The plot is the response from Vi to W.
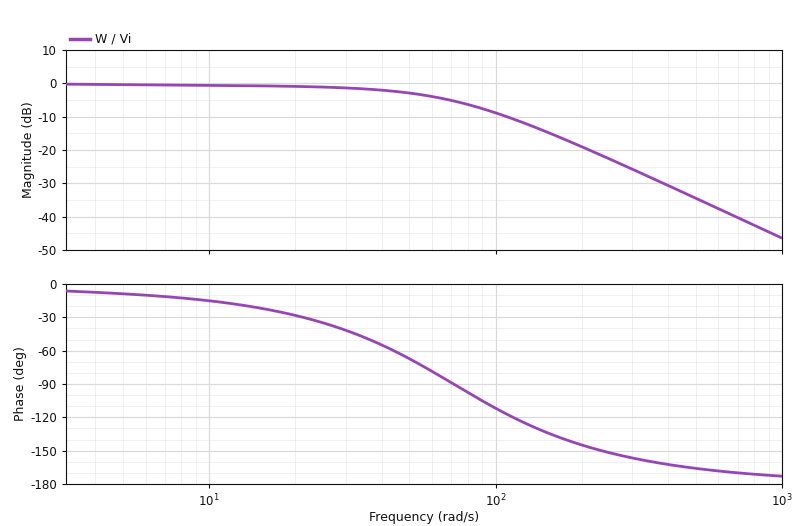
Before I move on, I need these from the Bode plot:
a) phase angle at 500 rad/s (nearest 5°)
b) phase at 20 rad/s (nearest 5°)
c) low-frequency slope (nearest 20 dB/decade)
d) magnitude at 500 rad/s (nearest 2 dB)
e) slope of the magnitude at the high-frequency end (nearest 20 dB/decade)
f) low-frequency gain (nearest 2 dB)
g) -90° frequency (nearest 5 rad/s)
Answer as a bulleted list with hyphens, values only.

- -165°
- -30°
- 0 dB/decade
- -34 dB
- -40 dB/decade
- 0 dB
- 70 rad/s
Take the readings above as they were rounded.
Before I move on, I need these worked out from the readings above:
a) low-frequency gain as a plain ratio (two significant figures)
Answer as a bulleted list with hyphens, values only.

- 1.0
